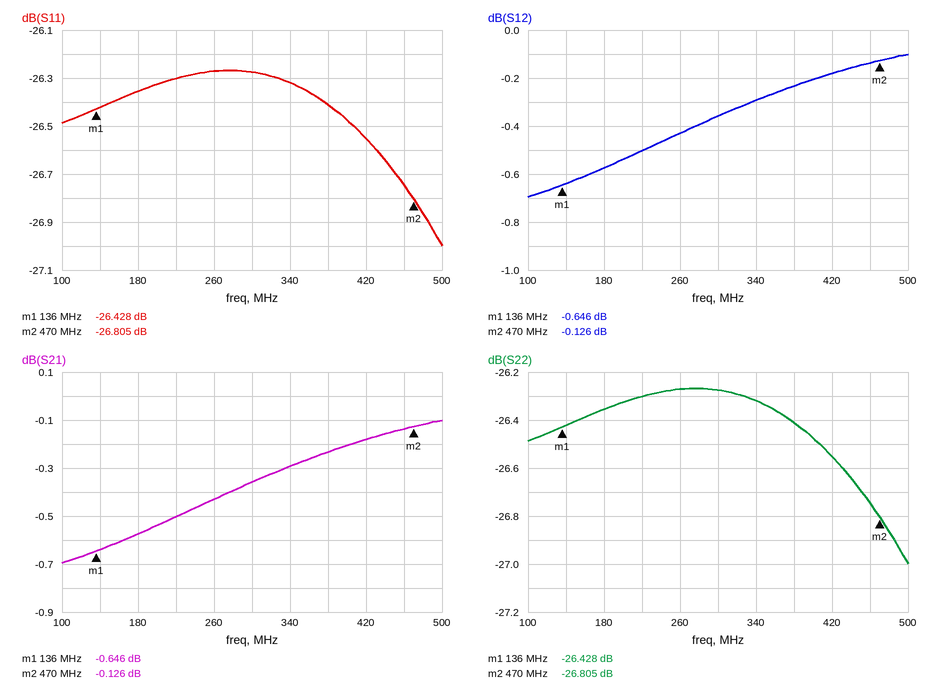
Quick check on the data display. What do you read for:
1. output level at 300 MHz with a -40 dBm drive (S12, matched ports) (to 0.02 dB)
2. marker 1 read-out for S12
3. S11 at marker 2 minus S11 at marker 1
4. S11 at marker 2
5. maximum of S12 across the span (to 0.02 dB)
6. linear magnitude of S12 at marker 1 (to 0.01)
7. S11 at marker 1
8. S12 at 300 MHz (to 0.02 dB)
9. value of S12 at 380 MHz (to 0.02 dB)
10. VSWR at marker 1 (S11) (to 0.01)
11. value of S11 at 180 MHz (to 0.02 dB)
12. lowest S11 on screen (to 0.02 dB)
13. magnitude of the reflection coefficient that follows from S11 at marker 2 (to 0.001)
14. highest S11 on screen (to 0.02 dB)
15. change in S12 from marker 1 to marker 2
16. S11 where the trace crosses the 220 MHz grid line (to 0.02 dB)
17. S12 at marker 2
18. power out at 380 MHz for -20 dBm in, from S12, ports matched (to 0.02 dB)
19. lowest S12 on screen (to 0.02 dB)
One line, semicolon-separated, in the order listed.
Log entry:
-40.36 dBm; -0.646 dB; -0.377 dB; -26.805 dB; -0.10 dB; 0.93; -26.428 dB; -0.36 dB; -0.24 dB; 1.10; -26.36 dB; -27.00 dB; 0.046; -26.26 dB; 0.520 dB; -26.30 dB; -0.126 dB; -20.24 dBm; -0.70 dB
